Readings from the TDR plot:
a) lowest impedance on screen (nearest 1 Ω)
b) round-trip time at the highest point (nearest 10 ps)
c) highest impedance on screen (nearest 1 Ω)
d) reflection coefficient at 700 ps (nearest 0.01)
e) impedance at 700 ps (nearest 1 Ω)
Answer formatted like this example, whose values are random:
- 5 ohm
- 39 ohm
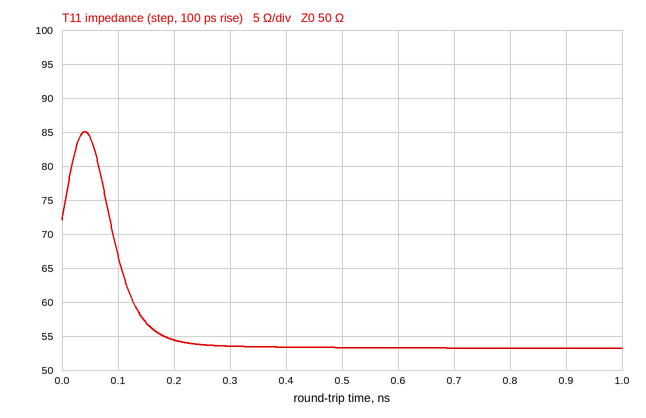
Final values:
- 53 Ω
- 40 ps
- 85 Ω
- +0.03
- 53 Ω
